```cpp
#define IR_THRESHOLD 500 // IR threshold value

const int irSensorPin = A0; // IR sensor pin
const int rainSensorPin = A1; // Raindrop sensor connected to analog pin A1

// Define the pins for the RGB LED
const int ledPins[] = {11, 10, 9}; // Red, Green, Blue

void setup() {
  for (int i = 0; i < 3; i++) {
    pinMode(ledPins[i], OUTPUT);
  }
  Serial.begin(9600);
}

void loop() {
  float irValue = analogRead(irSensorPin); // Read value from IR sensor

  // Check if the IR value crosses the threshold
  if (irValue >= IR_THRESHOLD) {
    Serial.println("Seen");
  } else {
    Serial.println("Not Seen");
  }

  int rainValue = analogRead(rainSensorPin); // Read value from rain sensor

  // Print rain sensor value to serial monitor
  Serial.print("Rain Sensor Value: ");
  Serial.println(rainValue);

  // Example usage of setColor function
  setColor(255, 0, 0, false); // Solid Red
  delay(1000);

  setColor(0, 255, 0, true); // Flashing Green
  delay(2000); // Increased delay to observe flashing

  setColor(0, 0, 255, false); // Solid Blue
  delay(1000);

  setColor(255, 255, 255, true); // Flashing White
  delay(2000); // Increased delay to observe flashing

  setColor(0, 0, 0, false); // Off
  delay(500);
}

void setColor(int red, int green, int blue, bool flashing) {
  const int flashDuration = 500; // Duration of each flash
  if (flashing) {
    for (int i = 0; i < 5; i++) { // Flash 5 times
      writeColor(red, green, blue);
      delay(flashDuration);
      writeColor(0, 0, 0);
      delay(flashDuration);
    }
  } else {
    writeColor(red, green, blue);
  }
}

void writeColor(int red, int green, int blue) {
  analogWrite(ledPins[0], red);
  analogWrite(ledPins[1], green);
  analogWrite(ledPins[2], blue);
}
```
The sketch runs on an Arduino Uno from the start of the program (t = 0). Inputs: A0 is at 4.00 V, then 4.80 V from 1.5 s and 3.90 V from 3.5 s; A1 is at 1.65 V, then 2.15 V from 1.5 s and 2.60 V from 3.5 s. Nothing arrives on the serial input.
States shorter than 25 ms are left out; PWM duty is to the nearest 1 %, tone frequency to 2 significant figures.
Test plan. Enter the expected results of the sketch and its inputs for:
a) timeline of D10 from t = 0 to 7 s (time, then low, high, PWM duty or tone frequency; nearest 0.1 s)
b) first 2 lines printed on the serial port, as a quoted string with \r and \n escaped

0 s low; 1 s high; 1.5 s low; 2 s high; 2.5 s low; 3 s high; 3.5 s low; 4 s high; 4.5 s low; 5 s high; 5.5 s low
"Seen\r\nRain Sensor Value: 337\r\n"
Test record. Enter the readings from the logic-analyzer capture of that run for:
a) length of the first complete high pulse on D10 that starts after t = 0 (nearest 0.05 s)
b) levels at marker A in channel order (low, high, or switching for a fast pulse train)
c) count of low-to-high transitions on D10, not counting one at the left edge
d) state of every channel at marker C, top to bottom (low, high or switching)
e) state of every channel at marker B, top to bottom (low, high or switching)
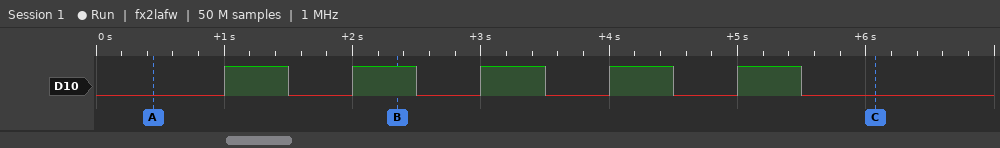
0.50 s
D10 low
5
D10 low
D10 high
